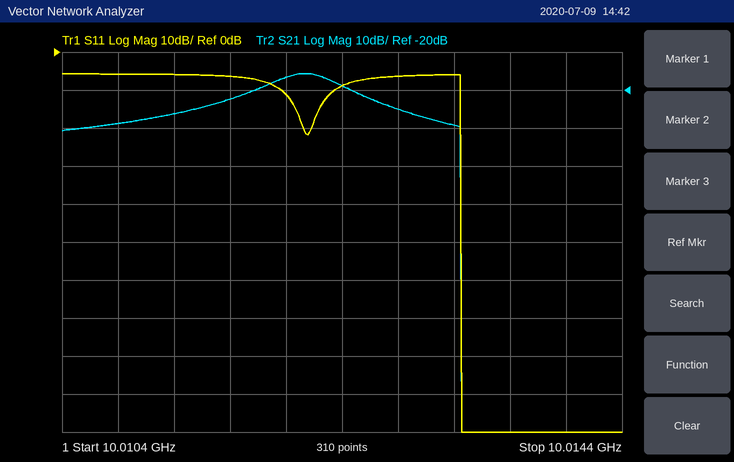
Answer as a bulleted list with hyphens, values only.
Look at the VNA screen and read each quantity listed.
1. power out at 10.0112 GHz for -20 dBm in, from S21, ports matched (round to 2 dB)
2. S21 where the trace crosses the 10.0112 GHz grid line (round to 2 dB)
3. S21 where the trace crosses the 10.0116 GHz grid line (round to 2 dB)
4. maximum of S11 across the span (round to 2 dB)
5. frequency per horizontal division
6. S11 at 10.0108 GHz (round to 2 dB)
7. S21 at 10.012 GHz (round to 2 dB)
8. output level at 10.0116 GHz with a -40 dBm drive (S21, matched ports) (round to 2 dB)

- -46 dBm
- -26 dB
- -22 dB
- -6 dB
- 400 kHz
- -6 dB
- -16 dB
- -62 dBm
